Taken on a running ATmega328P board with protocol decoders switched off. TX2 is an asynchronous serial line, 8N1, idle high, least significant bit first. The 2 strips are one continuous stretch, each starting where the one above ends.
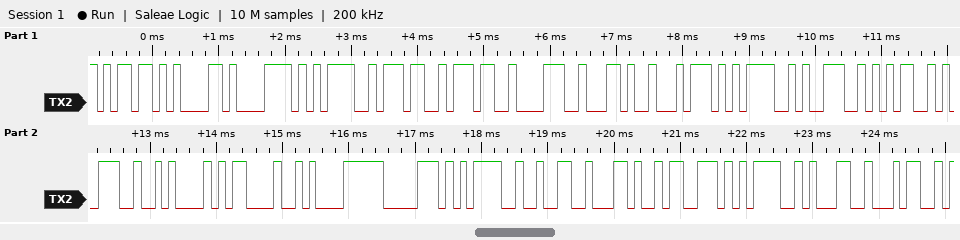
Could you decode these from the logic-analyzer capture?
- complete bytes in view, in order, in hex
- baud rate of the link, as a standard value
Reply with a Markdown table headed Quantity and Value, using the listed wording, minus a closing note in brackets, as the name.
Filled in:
| Quantity | Value |
|---|---|
| complete bytes in view, in order, in hex | 6D 61 78 3D 37 37 38 2C 74 3D 39 35 39 0A 0D 0A 70 3D 32 2C 73 3D 31 34 |
| baud rate of the link, as a standard value | 9600 baud |
